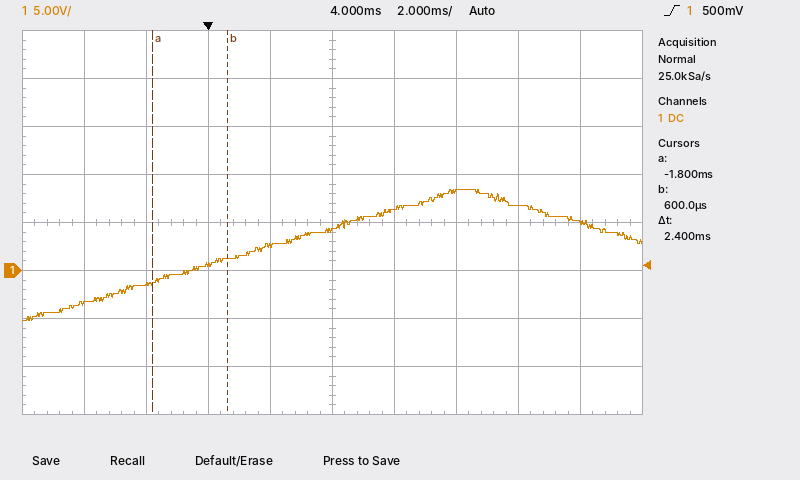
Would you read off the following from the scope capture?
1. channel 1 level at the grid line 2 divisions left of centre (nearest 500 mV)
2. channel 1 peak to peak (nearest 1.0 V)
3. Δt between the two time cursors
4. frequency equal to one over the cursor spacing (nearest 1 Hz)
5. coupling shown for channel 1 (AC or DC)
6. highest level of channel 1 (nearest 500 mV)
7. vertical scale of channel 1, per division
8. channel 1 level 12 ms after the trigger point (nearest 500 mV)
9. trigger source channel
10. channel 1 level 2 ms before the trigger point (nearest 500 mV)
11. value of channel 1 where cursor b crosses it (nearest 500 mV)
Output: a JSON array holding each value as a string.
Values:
["500 mV", "14.0 V", "2.4 ms", "417 Hz", "DC", "8.5 V", "5 V", "5.0 V", "channel 1", "-1.5 V", "1.0 V"]
